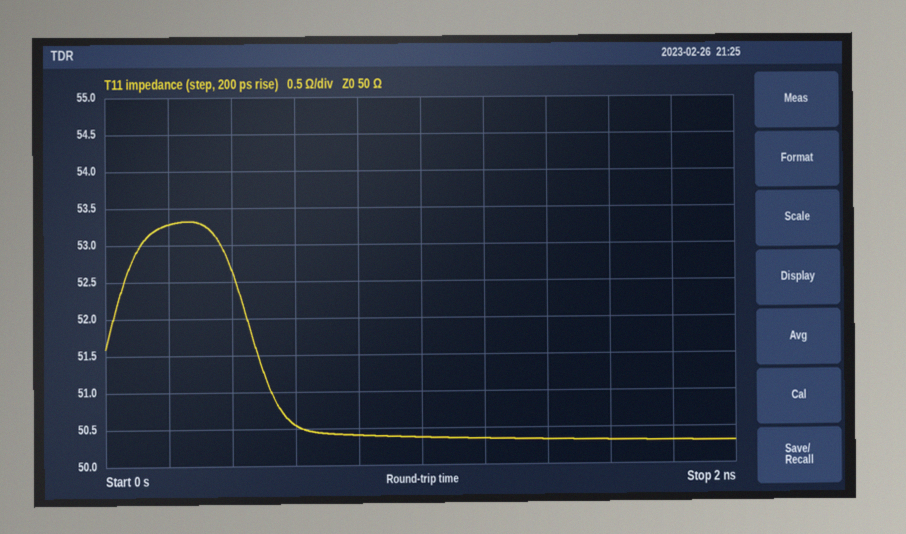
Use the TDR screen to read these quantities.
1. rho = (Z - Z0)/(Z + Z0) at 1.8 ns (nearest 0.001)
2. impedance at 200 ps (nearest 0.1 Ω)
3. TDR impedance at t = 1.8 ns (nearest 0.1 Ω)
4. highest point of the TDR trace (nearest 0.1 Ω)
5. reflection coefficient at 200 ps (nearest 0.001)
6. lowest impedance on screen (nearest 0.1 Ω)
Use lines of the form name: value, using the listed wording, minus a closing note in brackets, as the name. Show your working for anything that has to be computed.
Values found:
rho = (Z - Z0)/(Z + Z0) at 1.8 ns: (50.3 − 50)/(50.3 + 50) ≈ +0.003
impedance at 200 ps: 53.3 Ω
TDR impedance at t = 1.8 ns: 50.3 Ω
highest point of the TDR trace: 53.3 Ω
reflection coefficient at 200 ps: (53.3 − 50)/(53.3 + 50) ≈ +0.032
lowest impedance on screen: 50.3 Ω
